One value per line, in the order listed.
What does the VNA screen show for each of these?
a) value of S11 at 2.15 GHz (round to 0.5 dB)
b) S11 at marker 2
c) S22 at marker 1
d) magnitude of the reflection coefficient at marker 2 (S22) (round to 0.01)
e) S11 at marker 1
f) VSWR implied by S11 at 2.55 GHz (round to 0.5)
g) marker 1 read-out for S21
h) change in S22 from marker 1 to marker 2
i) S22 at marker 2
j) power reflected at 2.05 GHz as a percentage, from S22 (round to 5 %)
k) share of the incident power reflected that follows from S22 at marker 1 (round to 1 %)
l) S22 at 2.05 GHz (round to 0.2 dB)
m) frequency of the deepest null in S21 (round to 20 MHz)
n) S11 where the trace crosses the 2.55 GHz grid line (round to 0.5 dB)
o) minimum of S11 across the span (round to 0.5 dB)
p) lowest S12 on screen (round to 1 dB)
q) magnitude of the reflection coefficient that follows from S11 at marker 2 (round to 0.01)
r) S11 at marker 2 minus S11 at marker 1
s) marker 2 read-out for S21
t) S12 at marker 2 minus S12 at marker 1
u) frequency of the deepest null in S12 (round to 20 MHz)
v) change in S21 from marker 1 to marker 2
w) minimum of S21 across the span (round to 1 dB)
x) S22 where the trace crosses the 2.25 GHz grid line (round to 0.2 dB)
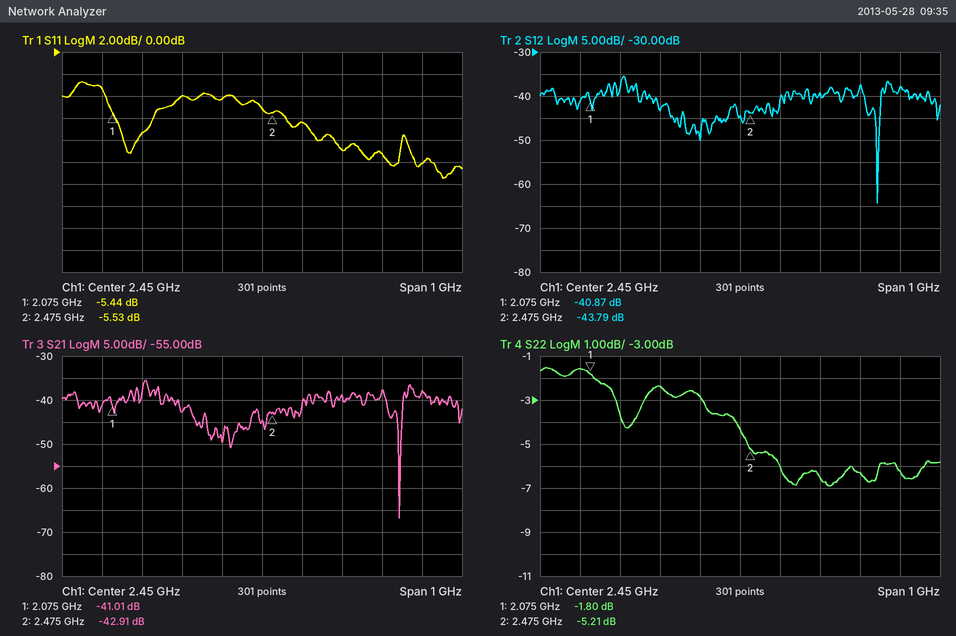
-7.5 dB
-5.53 dB
-1.80 dB
0.55
-5.44 dB
3.0
-41.01 dB
-3.41 dB
-5.21 dB
70 %
66 %
-1.6 dB
2.80 GHz
-6.5 dB
-11.5 dB
-64 dB
0.53
-0.09 dB
-42.91 dB
-2.92 dB
2.80 GHz
-1.90 dB
-67 dB
-2.4 dB
